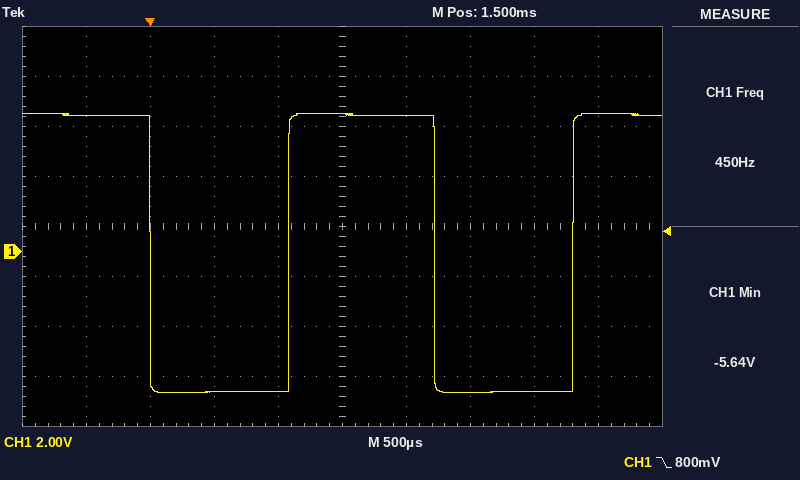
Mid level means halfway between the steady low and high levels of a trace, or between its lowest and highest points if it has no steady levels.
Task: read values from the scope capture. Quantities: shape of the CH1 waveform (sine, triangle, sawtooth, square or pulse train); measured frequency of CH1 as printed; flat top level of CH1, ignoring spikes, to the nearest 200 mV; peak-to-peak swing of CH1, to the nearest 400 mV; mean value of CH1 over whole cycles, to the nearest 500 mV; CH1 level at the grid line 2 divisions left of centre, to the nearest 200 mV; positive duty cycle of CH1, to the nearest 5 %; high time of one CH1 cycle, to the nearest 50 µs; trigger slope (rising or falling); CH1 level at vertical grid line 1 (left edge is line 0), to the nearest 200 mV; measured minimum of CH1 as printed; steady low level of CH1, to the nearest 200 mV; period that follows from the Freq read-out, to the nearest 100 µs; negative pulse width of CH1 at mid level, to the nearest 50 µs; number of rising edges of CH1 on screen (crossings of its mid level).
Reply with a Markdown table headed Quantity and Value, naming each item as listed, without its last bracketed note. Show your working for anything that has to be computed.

| Quantity | Value |
|---|---|
| shape of the CH1 waveform | square |
| measured frequency of CH1 as printed | 450 Hz |
| flat top level of CH1, ignoring spikes, to the nearest 200 mV | 5.4 V |
| peak-to-peak swing of CH1, to the nearest 400 mV | 11.2 V |
| mean value of CH1 over whole cycles, to the nearest 500 mV | -5.6 V + 0.5 × (5.4 V − (-5.6 V)) ≈ 0.0 V |
| CH1 level at the grid line 2 divisions left of centre, to the nearest 200 mV | -5.6 V |
| positive duty cycle of CH1, to the nearest 5 % | 50 % |
| high time of one CH1 cycle, to the nearest 50 µs | 1.15 ms |
| trigger slope | falling |
| CH1 level at vertical grid line 1 (left edge is line 0), to the nearest 200 mV | 5.4 V |
| measured minimum of CH1 as printed | -5.64 V |
| steady low level of CH1, to the nearest 200 mV | -5.6 V |
| period that follows from the Freq read-out, to the nearest 100 µs | 1 / 450 Hz ≈ 2.2 ms |
| negative pulse width of CH1 at mid level, to the nearest 50 µs | 1.10 ms |
| number of rising edges of CH1 on screen | 2 |
